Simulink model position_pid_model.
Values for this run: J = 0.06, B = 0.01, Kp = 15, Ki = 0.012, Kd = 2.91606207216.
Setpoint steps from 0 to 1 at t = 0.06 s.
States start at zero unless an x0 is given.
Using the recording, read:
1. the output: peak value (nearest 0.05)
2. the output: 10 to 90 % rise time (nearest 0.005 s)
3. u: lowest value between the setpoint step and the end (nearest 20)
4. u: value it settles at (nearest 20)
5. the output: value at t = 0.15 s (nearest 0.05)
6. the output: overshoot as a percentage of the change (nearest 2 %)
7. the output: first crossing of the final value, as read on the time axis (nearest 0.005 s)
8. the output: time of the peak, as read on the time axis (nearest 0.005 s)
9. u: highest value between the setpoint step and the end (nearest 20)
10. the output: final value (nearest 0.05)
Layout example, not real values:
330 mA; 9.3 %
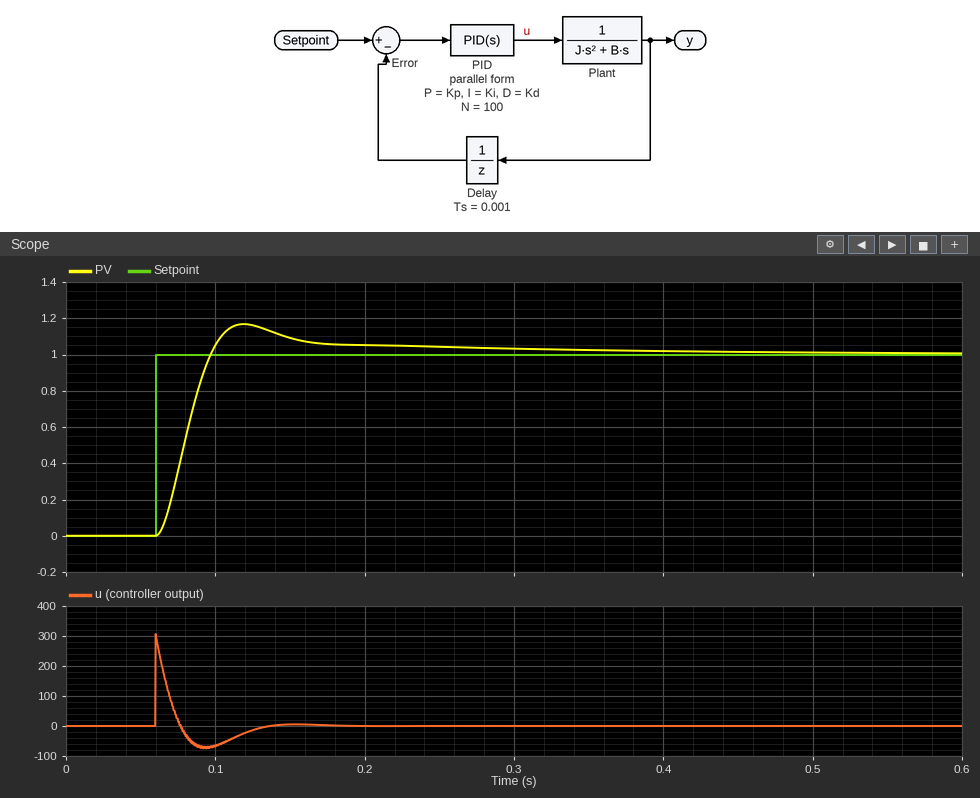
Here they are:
1.15; 0.025 s; -80; 0; 1.10; 16 %; 0.095 s; 0.120 s; 300; 1.00
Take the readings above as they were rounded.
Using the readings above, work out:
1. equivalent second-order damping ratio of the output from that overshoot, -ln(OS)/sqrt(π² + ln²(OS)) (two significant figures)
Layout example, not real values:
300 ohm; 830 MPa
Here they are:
0.50
